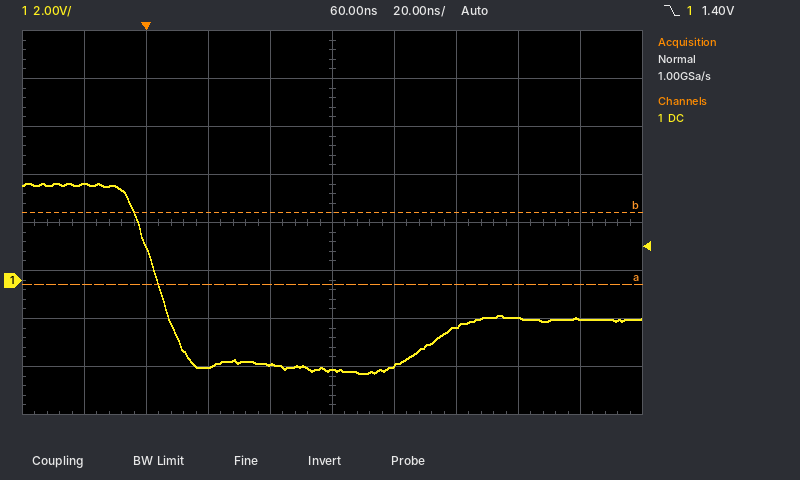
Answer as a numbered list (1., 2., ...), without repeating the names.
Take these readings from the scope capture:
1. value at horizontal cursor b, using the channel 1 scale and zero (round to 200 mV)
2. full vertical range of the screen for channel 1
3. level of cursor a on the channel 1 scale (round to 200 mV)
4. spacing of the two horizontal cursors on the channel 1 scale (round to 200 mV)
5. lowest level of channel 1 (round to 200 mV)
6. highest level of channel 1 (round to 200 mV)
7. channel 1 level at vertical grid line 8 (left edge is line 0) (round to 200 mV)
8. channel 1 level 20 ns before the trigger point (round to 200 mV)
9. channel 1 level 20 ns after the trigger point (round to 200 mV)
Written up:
1. 2.8 V
2. 16 V
3. -200 mV
4. 3.0 V
5. -3.8 V
6. 4.0 V
7. -1.6 V
8. 4.0 V
9. -3.6 V
